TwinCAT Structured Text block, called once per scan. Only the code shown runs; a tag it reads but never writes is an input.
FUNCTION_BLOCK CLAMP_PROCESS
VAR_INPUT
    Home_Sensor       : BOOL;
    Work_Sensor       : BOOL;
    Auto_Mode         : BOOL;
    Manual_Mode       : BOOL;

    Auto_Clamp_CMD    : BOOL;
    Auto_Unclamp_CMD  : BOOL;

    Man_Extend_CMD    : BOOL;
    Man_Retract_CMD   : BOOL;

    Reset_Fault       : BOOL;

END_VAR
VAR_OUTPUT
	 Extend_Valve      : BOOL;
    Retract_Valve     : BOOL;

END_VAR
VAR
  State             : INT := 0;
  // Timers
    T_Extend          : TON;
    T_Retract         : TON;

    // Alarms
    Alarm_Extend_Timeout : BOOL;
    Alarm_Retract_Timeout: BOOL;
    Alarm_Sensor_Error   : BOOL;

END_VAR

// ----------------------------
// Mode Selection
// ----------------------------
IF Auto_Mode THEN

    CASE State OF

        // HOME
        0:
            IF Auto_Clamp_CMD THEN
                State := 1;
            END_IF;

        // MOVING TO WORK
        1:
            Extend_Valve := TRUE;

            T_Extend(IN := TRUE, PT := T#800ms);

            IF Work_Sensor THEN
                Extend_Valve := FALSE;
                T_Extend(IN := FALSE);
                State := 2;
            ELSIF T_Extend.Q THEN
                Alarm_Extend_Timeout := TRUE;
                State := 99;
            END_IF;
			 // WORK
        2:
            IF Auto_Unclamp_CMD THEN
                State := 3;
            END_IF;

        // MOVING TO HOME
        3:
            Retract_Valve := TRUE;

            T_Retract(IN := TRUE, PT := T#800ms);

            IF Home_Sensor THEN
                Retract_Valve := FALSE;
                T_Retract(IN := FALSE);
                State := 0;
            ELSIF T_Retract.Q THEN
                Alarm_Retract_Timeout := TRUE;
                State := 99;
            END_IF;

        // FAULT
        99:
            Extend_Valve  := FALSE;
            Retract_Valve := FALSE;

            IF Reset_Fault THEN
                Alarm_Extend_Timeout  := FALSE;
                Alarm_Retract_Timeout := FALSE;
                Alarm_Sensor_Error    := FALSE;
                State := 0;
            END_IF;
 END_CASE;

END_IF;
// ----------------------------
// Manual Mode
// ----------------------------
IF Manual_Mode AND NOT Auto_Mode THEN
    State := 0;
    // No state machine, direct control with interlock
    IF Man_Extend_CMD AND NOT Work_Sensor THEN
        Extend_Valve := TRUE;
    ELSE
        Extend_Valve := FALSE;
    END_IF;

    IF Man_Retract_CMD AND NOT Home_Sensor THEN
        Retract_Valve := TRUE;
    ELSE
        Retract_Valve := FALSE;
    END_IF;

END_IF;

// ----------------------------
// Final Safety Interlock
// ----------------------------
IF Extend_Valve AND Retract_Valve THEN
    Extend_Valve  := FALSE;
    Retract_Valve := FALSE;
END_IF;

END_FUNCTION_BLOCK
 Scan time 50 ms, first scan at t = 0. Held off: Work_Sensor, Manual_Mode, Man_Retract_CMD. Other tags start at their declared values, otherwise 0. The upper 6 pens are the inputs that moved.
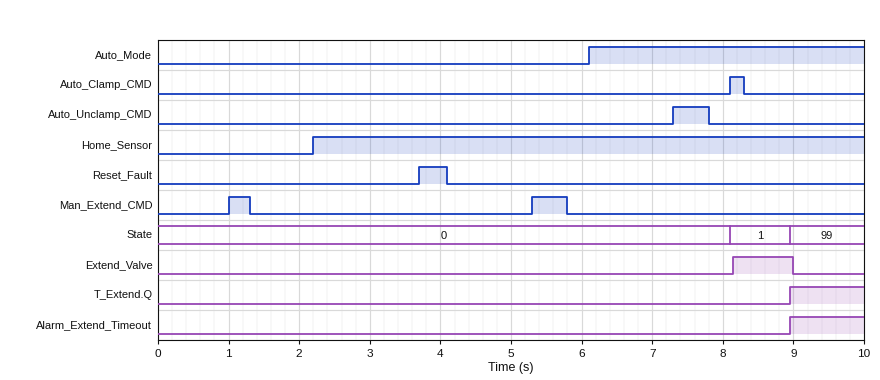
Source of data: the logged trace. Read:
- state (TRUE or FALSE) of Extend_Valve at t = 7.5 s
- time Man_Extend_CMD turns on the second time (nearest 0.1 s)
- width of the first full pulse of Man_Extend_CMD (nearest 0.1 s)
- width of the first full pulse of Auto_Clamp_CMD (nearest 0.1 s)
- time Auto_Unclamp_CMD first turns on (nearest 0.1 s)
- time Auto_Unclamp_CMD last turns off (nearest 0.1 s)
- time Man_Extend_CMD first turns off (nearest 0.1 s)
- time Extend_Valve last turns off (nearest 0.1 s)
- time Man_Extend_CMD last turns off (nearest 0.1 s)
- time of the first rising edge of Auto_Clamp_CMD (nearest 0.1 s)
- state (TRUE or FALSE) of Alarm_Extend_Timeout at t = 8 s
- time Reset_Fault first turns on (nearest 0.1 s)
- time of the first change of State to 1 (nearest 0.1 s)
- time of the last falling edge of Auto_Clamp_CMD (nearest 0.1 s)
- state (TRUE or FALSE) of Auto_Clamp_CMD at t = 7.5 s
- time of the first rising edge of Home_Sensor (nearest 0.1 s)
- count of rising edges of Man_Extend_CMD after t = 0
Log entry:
FALSE
5.3 s
0.3 s
0.2 s
7.3 s
7.8 s
1.3 s
9.0 s
5.8 s
8.1 s
FALSE
3.7 s
8.1 s
8.3 s
FALSE
2.2 s
2
